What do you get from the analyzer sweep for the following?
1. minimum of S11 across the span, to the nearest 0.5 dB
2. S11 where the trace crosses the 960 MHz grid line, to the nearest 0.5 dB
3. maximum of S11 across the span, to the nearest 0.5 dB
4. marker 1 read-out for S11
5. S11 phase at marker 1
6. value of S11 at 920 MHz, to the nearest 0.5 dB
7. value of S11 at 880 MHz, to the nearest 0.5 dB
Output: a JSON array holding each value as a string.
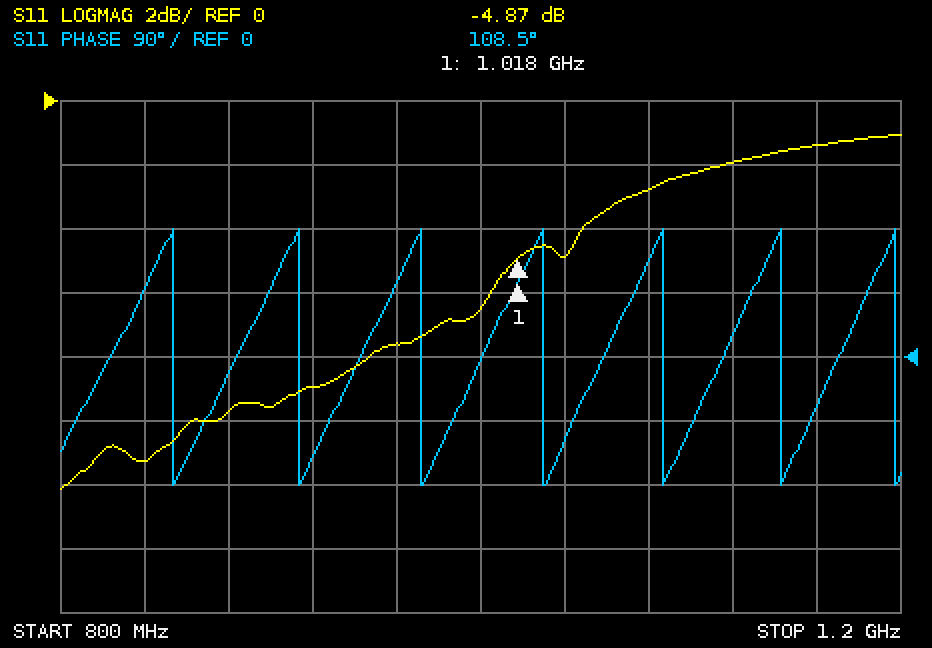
["-12.0 dB", "-7.5 dB", "-1.0 dB", "-4.87 dB", "108.5°", "-9.0 dB", "-9.5 dB"]
